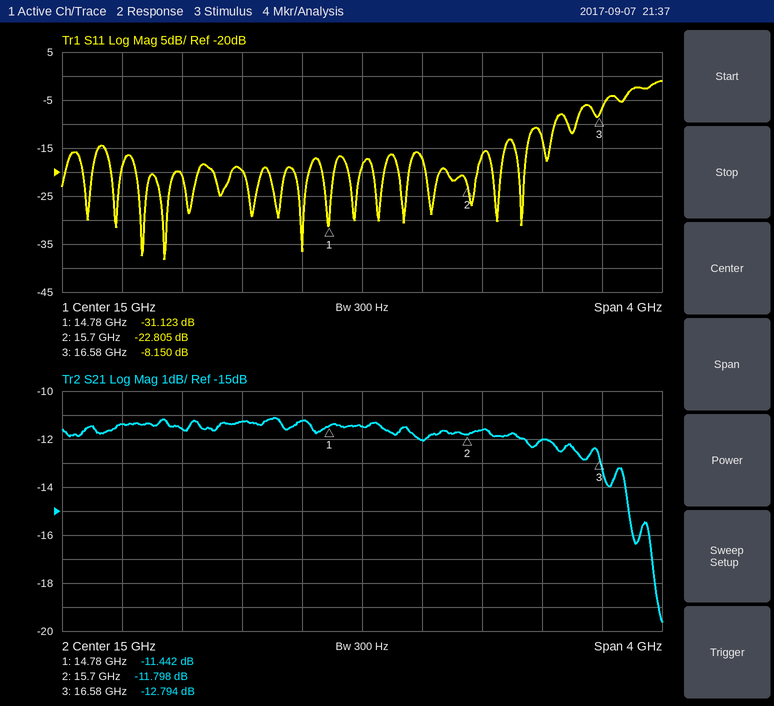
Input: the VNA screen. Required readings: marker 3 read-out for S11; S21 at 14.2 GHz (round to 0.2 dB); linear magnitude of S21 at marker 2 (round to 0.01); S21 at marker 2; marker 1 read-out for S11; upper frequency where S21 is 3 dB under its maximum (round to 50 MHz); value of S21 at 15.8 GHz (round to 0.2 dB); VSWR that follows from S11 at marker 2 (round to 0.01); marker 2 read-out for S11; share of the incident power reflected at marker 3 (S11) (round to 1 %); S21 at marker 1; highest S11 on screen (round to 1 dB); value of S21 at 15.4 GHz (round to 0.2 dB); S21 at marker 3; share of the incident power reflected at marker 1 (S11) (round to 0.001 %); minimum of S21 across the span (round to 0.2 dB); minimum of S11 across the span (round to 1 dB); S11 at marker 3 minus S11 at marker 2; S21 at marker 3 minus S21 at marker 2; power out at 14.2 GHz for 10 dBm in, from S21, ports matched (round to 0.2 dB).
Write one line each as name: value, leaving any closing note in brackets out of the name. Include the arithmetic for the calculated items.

marker 3 read-out for S11: -8.150 dB
S21 at 14.2 GHz: -11.2 dB
linear magnitude of S21 at marker 2: 10^(-11.798/20) ≈ 0.26
S21 at marker 2: -11.798 dB
marker 1 read-out for S11: -31.123 dB
upper frequency where S21 is 3 dB under its maximum: 16.75 GHz
value of S21 at 15.8 GHz: -11.6 dB
VSWR that follows from S11 at marker 2: (1 + 0.0724)/(1 − 0.0724) ≈ 1.16
marker 2 read-out for S11: -22.805 dB
share of the incident power reflected at marker 3 (S11): 10^(-8.15/10) ≈ 15 %
S21 at marker 1: -11.442 dB
highest S11 on screen: -1 dB
value of S21 at 15.4 GHz: -12.0 dB
S21 at marker 3: -12.794 dB
share of the incident power reflected at marker 1 (S11): 10^(-31.123/10) ≈ 0.077 %
minimum of S21 across the span: -19.6 dB
minimum of S11 across the span: -38 dB
S11 at marker 3 minus S11 at marker 2: -8.15 − (-22.805) = 14.655 dB
S21 at marker 3 minus S21 at marker 2: -12.794 − (-11.798) = -0.996 dB
power out at 14.2 GHz for 10 dBm in, from S21, ports matched: 10 dBm + (-11.2 dB) = -1.2 dBm
